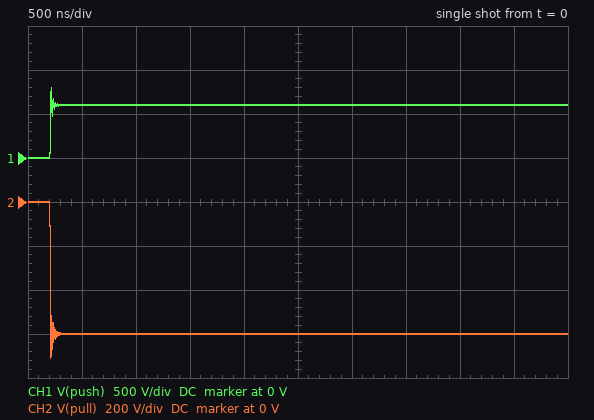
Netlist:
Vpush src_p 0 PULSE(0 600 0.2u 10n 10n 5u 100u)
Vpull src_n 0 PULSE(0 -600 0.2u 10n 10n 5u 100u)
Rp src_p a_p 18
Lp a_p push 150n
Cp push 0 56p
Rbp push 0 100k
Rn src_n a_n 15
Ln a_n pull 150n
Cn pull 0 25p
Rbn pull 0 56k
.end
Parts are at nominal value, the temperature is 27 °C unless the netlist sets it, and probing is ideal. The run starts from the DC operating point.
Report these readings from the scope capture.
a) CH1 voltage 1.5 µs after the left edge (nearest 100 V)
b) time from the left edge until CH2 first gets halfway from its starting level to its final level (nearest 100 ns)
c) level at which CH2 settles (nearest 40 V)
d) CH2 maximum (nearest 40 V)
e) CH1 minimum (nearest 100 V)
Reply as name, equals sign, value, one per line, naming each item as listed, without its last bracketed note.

CH1 voltage 1.5 µs after the left edge = 600 V
time from the left edge until CH2 first gets halfway from its starting level to its final level = 200 ns
level at which CH2 settles = -600 V
CH2 maximum = 0 V
CH1 minimum = 0 V
